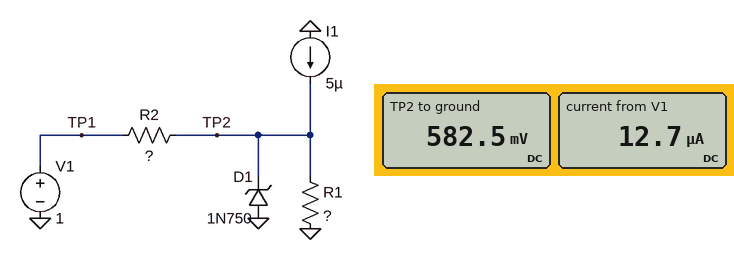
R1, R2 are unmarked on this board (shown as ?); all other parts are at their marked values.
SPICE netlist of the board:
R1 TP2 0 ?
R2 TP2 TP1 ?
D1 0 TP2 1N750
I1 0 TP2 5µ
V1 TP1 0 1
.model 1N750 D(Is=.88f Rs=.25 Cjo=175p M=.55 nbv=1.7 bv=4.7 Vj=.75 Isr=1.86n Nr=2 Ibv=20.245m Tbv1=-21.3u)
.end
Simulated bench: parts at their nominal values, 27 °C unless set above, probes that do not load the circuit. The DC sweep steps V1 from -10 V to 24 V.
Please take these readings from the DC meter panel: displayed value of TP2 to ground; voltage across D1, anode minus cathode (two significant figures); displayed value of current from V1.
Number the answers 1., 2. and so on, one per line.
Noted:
1. 582.5 mV
2. -580 mV
3. 12.7 µA
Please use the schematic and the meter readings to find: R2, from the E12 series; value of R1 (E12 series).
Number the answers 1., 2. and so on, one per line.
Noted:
1. 33 kΩ
2. 33 kΩ
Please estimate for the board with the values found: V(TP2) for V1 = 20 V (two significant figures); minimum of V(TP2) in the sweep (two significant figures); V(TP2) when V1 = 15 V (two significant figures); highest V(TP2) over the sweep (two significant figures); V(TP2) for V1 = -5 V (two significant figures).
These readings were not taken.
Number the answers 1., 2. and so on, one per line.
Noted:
1. 4.5 V
2. -650 mV
3. 4.5 V
4. 4.5 V
5. -610 mV
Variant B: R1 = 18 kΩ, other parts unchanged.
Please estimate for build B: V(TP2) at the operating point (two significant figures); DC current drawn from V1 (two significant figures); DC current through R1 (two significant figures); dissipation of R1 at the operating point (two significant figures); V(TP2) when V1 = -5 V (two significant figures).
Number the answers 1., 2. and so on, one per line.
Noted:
1. 410 mV
2. 18 µA
3. 23 µA
4. 9.4 µW
5. -600 mV
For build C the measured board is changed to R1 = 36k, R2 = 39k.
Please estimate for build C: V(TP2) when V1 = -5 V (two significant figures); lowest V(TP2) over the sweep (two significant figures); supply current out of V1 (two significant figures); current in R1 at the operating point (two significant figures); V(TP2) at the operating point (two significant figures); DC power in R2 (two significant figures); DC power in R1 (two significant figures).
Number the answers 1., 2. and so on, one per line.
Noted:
1. -600 mV
2. -640 mV
3. 11 µA
4. 16 µA
5. 570 mV
6. 4.7 µW
7. 9.1 µW
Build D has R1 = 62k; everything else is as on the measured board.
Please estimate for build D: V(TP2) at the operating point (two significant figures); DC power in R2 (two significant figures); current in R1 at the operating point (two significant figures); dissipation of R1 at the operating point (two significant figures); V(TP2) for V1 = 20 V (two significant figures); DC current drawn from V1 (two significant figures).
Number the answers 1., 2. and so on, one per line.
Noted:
1. 760 mV
2. 1.7 µW
3. 12 µA
4. 9.3 µW
5. 4.5 V
6. 7.3 µA
